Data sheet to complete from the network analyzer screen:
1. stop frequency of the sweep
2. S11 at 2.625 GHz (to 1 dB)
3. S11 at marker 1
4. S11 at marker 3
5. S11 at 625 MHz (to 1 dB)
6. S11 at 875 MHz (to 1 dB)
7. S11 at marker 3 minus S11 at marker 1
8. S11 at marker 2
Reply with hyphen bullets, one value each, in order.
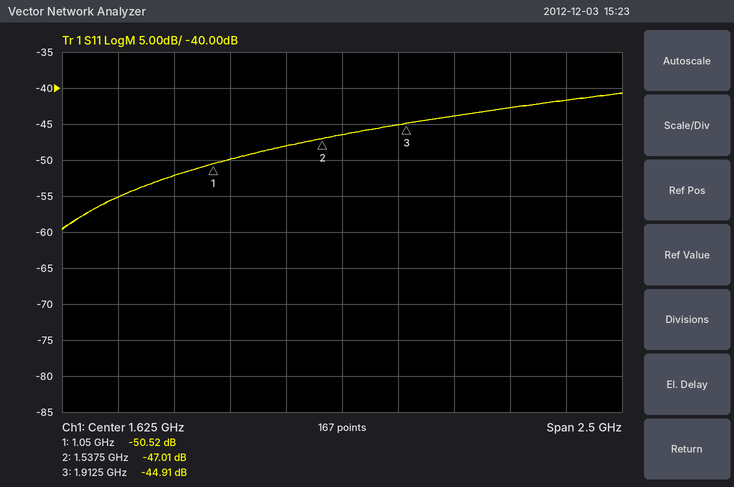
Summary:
- 2.875 GHz
- -42 dB
- -50.52 dB
- -44.91 dB
- -55 dB
- -52 dB
- 5.61 dB
- -47.01 dB
